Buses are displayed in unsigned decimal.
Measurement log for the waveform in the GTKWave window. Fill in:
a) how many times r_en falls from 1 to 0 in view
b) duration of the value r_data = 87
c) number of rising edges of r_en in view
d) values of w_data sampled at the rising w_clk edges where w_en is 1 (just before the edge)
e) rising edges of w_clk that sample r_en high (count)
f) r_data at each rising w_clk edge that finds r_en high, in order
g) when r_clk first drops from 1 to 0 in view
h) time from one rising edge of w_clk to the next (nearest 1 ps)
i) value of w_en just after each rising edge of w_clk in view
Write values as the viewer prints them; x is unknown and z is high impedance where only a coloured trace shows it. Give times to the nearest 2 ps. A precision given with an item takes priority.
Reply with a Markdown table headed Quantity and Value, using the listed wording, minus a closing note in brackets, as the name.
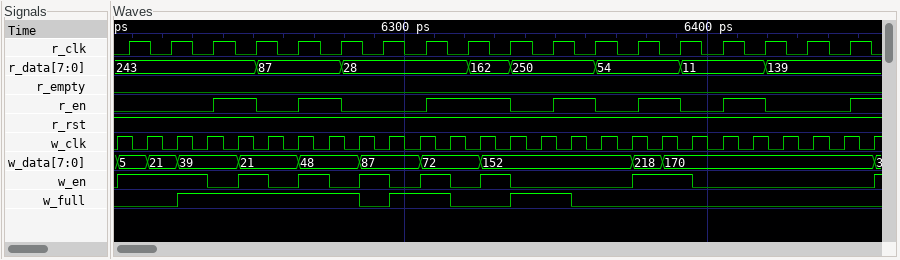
| Quantity | Value |
|---|---|
| how many times r_en falls from 1 to 0 in view | 6 |
| duration of the value r_data = 87 | 28 ps |
| number of rising edges of r_en in view | 7 |
| values of w_data sampled at the rising w_clk edges where w_en is 1 | 5, 21, 39, 21, 48, 87, 72, 152, 218, 170 |
| rising edges of w_clk that sample r_en high | 9 |
| r_data at each rising w_clk edge that finds r_en high, in order | 243, 87, 28, 162, 162, 250, 54, 11, 139 |
| when r_clk first drops from 1 to 0 in view | 6216 ps |
| time from one rising edge of w_clk to the next | 10 ps |
| value of w_en just after each rising edge of w_clk in view | 1 1 1 0 1 0 1 0 1 0 1 0 1 0 0 0 0 1 1 0 0 0 0 0 0 1 |
